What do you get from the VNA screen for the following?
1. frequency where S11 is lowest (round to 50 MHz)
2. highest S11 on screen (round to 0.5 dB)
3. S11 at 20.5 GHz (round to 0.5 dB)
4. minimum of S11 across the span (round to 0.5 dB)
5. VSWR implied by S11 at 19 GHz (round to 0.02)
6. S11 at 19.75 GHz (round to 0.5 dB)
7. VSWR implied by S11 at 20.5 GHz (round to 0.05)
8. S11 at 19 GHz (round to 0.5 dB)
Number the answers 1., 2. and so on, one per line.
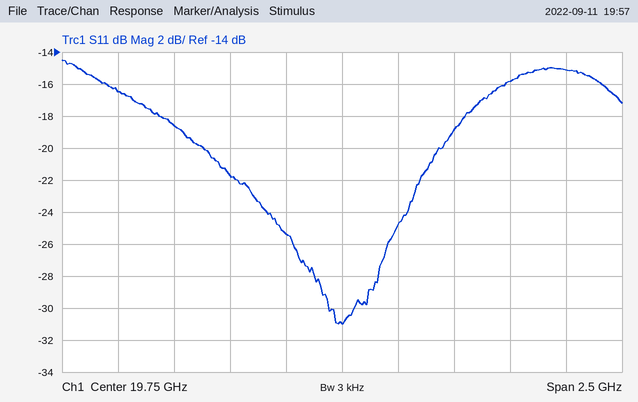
1. 19.75 GHz
2. -14.5 dB
3. -16.0 dB
4. -31.0 dB
5. 1.26
6. -31.0 dB
7. 1.40
8. -18.5 dB
